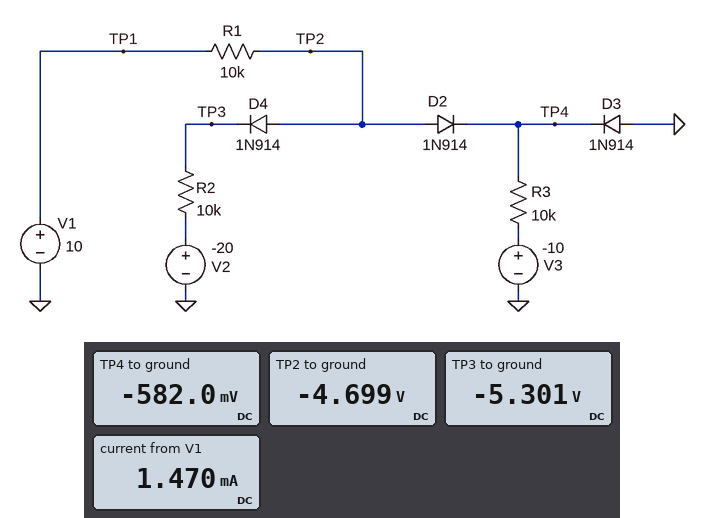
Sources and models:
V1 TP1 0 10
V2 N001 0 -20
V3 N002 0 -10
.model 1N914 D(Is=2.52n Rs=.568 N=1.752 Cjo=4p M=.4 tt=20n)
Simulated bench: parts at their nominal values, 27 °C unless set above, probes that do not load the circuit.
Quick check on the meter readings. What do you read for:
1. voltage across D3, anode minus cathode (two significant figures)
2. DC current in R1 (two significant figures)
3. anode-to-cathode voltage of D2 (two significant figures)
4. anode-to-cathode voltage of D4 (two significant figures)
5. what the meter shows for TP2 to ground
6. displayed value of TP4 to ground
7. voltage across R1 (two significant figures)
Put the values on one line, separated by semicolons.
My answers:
580 mV; 1.5 mA; -4.1 V; 600 mV; -4.699 V; -582.0 mV; 15 V
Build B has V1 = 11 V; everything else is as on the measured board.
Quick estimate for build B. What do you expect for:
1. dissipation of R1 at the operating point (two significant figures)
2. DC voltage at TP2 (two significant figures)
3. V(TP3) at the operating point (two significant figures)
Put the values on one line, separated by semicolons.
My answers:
23 mW; -4.2 V; -4.8 V
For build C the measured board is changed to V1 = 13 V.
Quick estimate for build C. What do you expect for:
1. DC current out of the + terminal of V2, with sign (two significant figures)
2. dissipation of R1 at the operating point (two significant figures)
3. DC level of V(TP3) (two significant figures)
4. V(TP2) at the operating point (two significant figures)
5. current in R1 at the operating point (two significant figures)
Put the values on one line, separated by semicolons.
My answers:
-1.6 mA; 26 mW; -3.8 V; -3.2 V; 1.6 mA
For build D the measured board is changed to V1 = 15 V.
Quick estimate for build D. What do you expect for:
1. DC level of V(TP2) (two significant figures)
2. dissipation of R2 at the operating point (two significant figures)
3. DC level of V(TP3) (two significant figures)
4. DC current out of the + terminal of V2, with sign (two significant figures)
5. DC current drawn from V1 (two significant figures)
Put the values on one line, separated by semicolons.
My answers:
-2.2 V; 30 mW; -2.8 V; -1.7 mA; 1.7 mA
